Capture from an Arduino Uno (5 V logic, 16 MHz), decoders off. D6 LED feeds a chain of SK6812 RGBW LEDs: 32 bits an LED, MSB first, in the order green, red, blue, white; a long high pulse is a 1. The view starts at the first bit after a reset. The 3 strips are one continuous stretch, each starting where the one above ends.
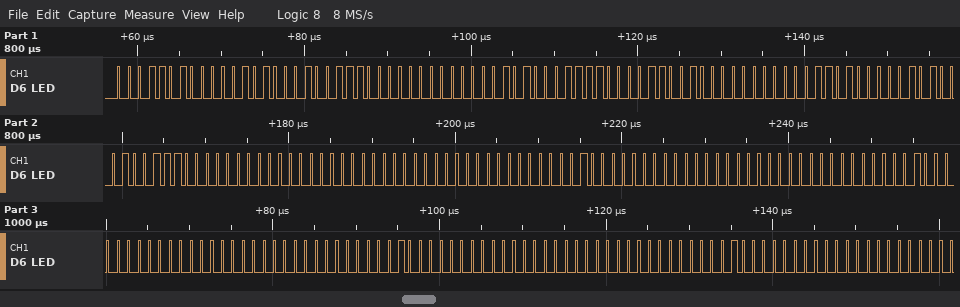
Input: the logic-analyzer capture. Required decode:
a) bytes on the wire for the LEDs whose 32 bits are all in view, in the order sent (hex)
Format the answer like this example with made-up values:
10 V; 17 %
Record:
1A 0A 27 00 05 1E 19 00 1A 0A 27 00 00 00 00 02 00 00 00 02 00 00 00 02 00 00 00 02
